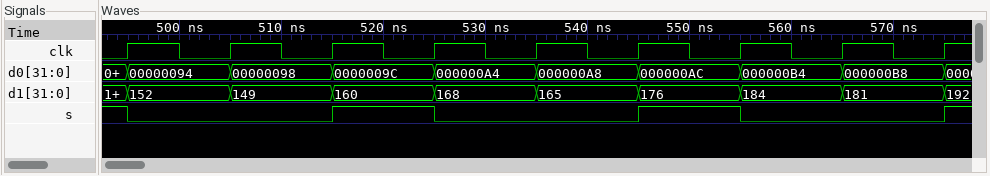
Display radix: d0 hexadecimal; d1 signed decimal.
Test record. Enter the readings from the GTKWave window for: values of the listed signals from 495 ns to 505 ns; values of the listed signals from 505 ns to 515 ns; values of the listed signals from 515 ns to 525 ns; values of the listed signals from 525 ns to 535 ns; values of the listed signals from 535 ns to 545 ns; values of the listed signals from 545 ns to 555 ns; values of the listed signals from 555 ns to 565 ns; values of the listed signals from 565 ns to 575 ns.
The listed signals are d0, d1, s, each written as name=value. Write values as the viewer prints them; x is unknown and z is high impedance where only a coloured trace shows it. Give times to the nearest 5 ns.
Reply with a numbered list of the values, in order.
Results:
1. d0=00000094, d1=152, s=0
2. d0=00000098, d1=149, s=0
3. d0=0000009C, d1=160, s=1
4. d0=000000A4, d1=168, s=0
5. d0=000000A8, d1=165, s=0
6. d0=000000AC, d1=176, s=1
7. d0=000000B4, d1=184, s=0
8. d0=000000B8, d1=181, s=0
